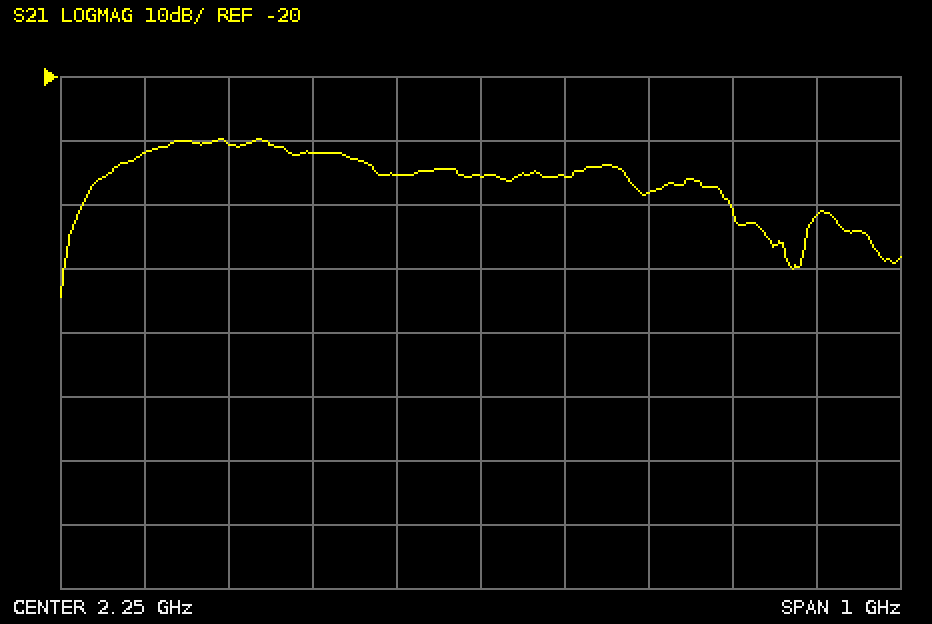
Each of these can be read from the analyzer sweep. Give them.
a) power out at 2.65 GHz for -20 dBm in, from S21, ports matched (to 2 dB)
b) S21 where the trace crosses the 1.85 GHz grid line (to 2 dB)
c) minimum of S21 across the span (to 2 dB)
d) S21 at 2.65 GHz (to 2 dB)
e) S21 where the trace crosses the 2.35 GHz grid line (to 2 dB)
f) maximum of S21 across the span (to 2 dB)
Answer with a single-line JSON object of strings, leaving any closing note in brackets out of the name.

{"power out at 2.65 GHz for -20 dBm in, from S21, ports matched": "-62 dBm", "S21 where the trace crosses the 1.85 GHz grid line": "-32 dB", "minimum of S21 across the span": "-54 dB", "S21 at 2.65 GHz": "-42 dB", "S21 where the trace crosses the 2.35 GHz grid line": "-36 dB", "maximum of S21 across the span": "-30 dB"}
